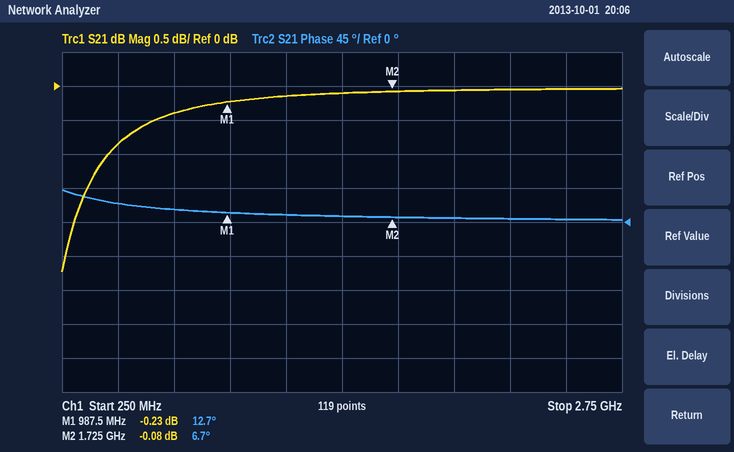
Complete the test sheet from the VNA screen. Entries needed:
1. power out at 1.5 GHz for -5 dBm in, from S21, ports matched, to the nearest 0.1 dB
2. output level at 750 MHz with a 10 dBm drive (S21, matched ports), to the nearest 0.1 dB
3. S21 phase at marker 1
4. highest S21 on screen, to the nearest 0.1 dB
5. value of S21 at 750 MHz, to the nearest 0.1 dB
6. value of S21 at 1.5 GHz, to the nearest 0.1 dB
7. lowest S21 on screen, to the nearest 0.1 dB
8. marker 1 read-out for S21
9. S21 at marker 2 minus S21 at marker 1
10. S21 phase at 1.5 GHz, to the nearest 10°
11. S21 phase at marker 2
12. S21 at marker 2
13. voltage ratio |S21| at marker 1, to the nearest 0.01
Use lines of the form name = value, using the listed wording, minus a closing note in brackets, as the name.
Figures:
power out at 1.5 GHz for -5 dBm in, from S21, ports matched, to the nearest 0.1 dB = -5.1 dBm
output level at 750 MHz with a 10 dBm drive (S21, matched ports), to the nearest 0.1 dB = 9.6 dBm
S21 phase at marker 1 = 12.7°
highest S21 on screen, to the nearest 0.1 dB = 0.0 dB
value of S21 at 750 MHz, to the nearest 0.1 dB = -0.4 dB
value of S21 at 1.5 GHz, to the nearest 0.1 dB = -0.1 dB
lowest S21 on screen, to the nearest 0.1 dB = -2.7 dB
marker 1 read-out for S21 = -0.23 dB
S21 at marker 2 minus S21 at marker 1 = 0.15 dB
S21 phase at 1.5 GHz, to the nearest 10° = 10°
S21 phase at marker 2 = 6.7°
S21 at marker 2 = -0.08 dB
voltage ratio |S21| at marker 1, to the nearest 0.01 = 0.97
